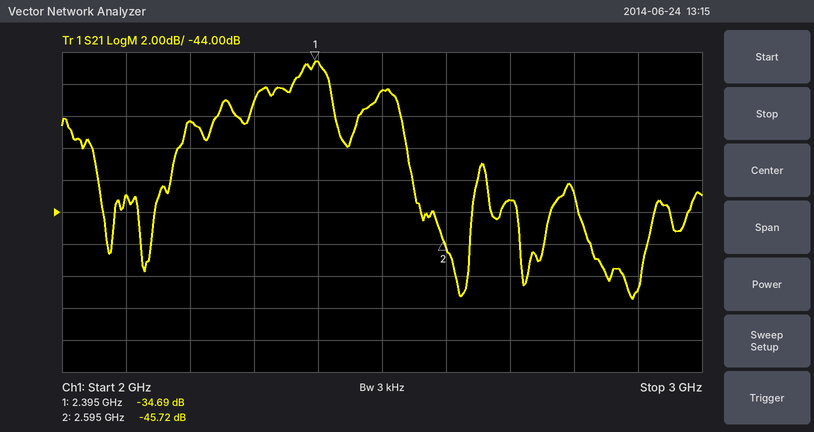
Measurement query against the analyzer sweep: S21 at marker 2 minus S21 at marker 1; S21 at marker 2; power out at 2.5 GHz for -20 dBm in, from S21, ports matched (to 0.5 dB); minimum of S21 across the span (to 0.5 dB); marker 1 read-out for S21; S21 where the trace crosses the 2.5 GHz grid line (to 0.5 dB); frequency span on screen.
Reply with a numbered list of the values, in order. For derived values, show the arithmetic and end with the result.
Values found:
1. -45.72 − (-34.69) = -11.03 dB
2. -45.72 dB
3. -20 dBm + (-36.5 dB) = -56.5 dBm
4. -49.5 dB
5. -34.69 dB
6. -36.5 dB
7. 1 GHz
